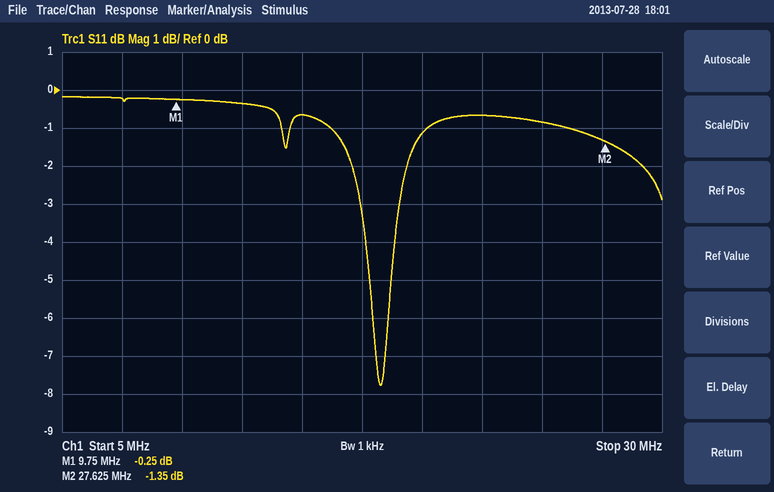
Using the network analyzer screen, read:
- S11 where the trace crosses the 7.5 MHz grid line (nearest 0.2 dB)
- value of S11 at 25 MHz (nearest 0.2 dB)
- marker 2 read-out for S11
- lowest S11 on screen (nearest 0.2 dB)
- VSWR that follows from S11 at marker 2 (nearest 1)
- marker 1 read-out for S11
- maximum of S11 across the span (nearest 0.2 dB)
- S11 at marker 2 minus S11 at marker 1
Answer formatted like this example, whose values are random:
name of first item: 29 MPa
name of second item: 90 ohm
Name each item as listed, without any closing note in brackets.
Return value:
S11 where the trace crosses the 7.5 MHz grid line: -0.2 dB
value of S11 at 25 MHz: -0.8 dB
marker 2 read-out for S11: -1.35 dB
lowest S11 on screen: -7.8 dB
VSWR that follows from S11 at marker 2: 13
marker 1 read-out for S11: -0.25 dB
maximum of S11 across the span: -0.2 dB
S11 at marker 2 minus S11 at marker 1: -1.10 dB
